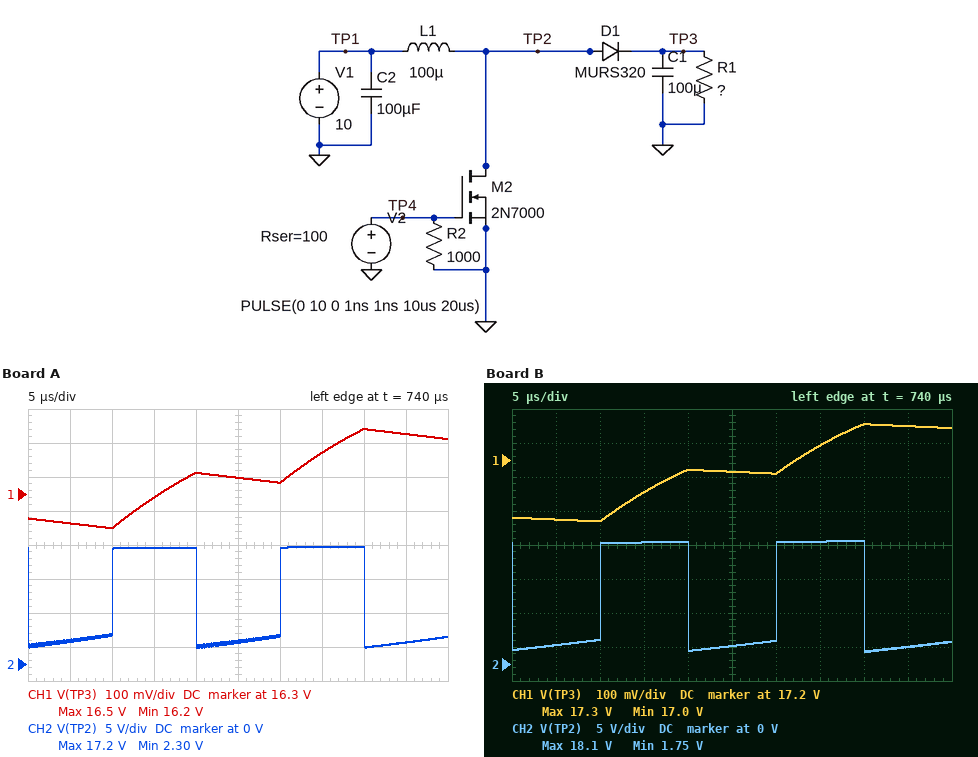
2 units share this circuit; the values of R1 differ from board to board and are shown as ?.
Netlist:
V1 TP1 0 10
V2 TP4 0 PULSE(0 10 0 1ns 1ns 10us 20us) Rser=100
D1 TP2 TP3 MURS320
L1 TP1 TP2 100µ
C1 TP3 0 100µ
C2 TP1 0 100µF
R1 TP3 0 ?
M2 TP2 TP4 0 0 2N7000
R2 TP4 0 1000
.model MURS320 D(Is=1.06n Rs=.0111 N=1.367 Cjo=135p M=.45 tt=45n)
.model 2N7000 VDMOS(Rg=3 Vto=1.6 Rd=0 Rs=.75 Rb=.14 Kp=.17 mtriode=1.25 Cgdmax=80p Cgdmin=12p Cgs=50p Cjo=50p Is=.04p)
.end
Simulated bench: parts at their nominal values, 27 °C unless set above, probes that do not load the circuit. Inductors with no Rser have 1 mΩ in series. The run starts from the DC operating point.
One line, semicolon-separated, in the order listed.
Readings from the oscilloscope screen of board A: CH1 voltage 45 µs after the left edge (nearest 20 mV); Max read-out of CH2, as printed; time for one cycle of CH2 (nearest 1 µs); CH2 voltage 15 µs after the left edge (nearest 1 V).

16.48 V; 17.2 V; 20 µs; 17 V
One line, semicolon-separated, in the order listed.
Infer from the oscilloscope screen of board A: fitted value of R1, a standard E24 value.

56 Ω
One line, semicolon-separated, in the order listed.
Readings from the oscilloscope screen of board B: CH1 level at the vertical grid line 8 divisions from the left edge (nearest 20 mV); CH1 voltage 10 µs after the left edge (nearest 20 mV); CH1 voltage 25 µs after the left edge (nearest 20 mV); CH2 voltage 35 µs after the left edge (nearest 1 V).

17.30 V; 17.02 V; 17.16 V; 18 V
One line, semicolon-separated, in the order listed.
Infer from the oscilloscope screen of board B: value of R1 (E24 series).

150 Ω
